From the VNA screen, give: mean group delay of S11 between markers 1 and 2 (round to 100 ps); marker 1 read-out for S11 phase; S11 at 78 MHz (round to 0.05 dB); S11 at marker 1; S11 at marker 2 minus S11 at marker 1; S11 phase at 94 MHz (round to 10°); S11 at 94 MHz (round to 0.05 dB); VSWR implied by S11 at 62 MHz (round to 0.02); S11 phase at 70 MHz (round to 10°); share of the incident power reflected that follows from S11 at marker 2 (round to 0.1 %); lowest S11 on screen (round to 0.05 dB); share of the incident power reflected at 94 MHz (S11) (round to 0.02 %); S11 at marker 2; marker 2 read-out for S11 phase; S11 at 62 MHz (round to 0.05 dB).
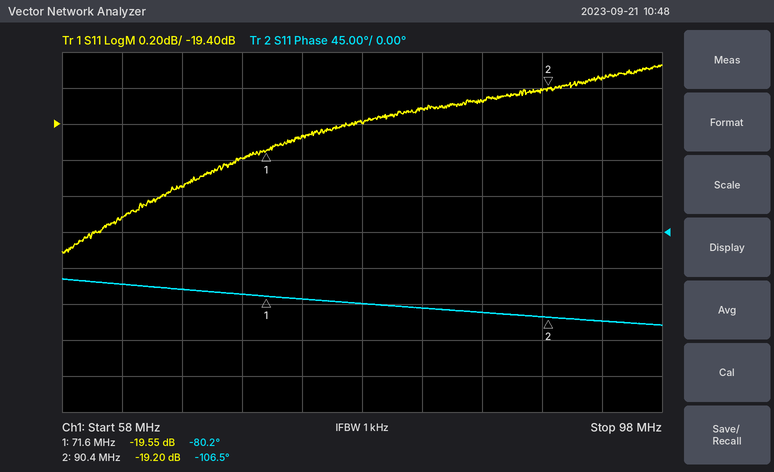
3.9 ns
-80.2°
-19.40 dB
-19.55 dB
0.35 dB
-110°
-19.15 dB
1.22
-80°
1.2 %
-20.10 dB
1.22 %
-19.20 dB
-106.5°
-19.90 dB
